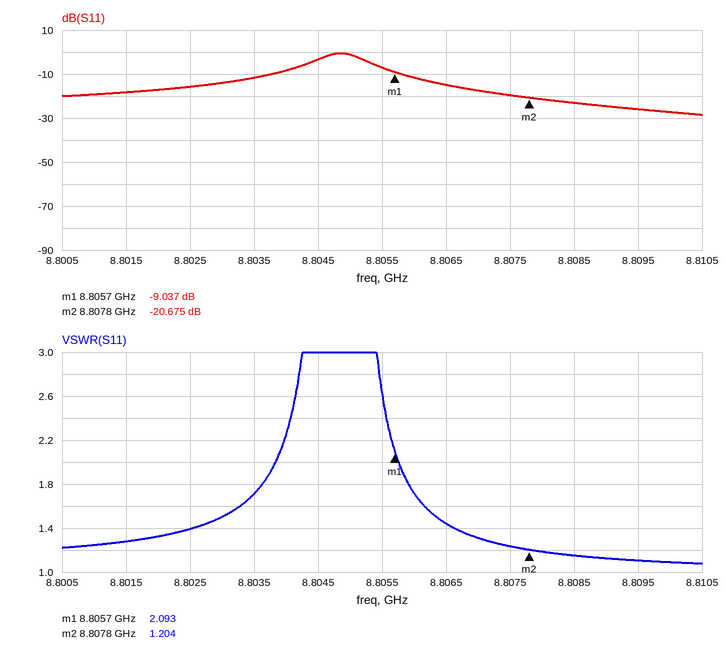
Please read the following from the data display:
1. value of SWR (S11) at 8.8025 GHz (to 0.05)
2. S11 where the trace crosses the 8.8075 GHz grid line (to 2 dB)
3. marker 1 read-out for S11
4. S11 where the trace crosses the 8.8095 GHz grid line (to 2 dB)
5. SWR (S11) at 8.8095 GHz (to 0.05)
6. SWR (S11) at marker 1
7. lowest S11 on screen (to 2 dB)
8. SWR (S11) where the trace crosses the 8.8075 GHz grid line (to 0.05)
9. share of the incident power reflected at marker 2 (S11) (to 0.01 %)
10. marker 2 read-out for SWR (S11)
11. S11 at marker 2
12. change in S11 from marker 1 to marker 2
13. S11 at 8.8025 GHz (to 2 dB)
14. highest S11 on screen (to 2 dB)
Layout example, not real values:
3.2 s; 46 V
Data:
1.40; -20 dB; -9.037 dB; -26 dB; 1.10; 2.093; -28 dB; 1.25; 0.86 %; 1.204; -20.675 dB; -11.638 dB; -16 dB; 0 dB
